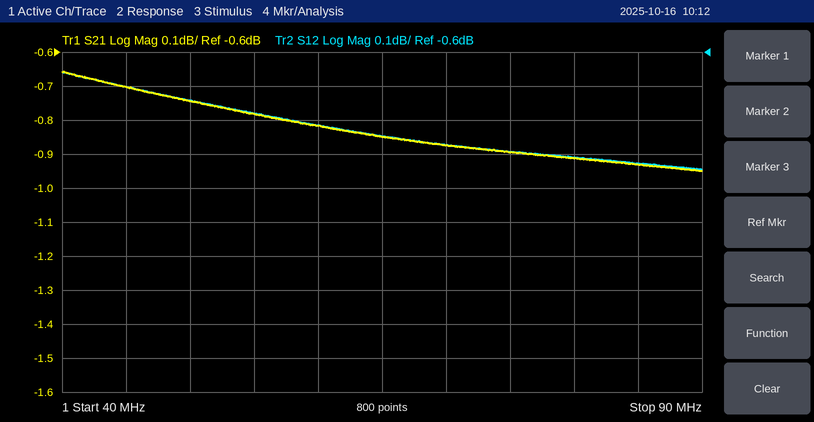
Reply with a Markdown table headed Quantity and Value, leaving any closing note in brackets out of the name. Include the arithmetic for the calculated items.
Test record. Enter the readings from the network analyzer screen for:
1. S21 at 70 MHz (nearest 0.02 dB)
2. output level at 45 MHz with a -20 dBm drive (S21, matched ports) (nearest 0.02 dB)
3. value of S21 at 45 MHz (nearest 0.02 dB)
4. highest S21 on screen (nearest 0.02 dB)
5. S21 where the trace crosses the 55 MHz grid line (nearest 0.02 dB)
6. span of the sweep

| Quantity | Value |
|---|---|
| S21 at 70 MHz | -0.88 dB |
| output level at 45 MHz with a -20 dBm drive (S21, matched ports) | -20 dBm + (-0.70 dB) = -20.70 dBm |
| value of S21 at 45 MHz | -0.70 dB |
| highest S21 on screen | -0.66 dB |
| S21 where the trace crosses the 55 MHz grid line | -0.78 dB |
| span of the sweep | 50 MHz |
